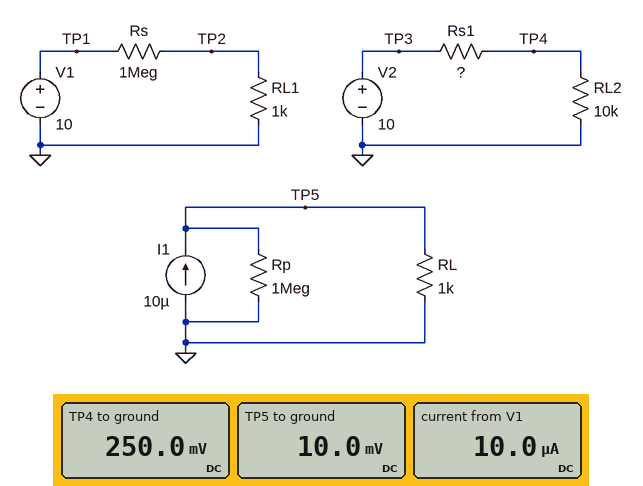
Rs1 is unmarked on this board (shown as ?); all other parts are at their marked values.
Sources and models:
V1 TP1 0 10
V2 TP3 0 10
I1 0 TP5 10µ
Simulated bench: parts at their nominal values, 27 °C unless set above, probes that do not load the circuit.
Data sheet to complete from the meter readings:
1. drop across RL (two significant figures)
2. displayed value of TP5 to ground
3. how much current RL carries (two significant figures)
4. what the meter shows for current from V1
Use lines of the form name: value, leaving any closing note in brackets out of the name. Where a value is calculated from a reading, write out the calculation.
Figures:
drop across RL: 10 mV = 10 mV
displayed value of TP5 to ground: 10.0 mV
how much current RL carries: (10 mV) / 1 kΩ = 10 µA
what the meter shows for current from V1: 10.0 µA
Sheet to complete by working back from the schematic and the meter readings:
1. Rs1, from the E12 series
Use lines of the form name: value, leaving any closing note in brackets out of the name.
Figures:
Rs1, from the E12 series: 390 kΩ
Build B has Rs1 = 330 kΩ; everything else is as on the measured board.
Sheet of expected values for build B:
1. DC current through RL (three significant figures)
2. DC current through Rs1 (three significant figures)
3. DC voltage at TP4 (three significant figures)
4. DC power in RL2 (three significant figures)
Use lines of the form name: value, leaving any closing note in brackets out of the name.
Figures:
DC current through RL: 9.99 µA
DC current through Rs1: 29.4 µA
DC voltage at TP4: 294 mV
DC power in RL2: 8.65 µW
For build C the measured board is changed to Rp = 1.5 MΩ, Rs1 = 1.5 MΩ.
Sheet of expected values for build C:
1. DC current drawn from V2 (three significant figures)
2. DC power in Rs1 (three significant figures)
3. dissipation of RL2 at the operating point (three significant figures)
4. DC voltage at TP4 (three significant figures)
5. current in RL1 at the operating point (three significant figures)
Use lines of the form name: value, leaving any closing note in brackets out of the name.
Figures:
DC current drawn from V2: 6.62 µA
DC power in Rs1: 65.8 µW
dissipation of RL2 at the operating point: 439 nW
DC voltage at TP4: 66.2 mV
current in RL1 at the operating point: 9.99 µA
